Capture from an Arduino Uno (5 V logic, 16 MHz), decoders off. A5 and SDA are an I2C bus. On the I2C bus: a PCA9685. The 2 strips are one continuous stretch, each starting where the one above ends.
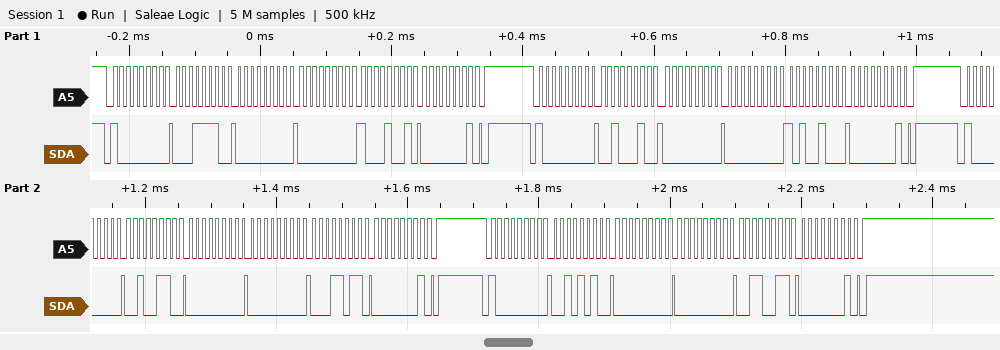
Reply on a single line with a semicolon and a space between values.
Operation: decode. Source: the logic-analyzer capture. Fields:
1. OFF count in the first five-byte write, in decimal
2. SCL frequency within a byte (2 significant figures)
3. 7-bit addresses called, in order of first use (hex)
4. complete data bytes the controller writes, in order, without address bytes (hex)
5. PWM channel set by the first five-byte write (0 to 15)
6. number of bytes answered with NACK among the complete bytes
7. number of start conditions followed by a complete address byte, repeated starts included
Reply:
393; 100 kHz; 0x40; 1E 00 00 89 01 22 00 00 A4 01 26 00 00 1B 01 2A 00 00 33 01; 6; 0; 4
